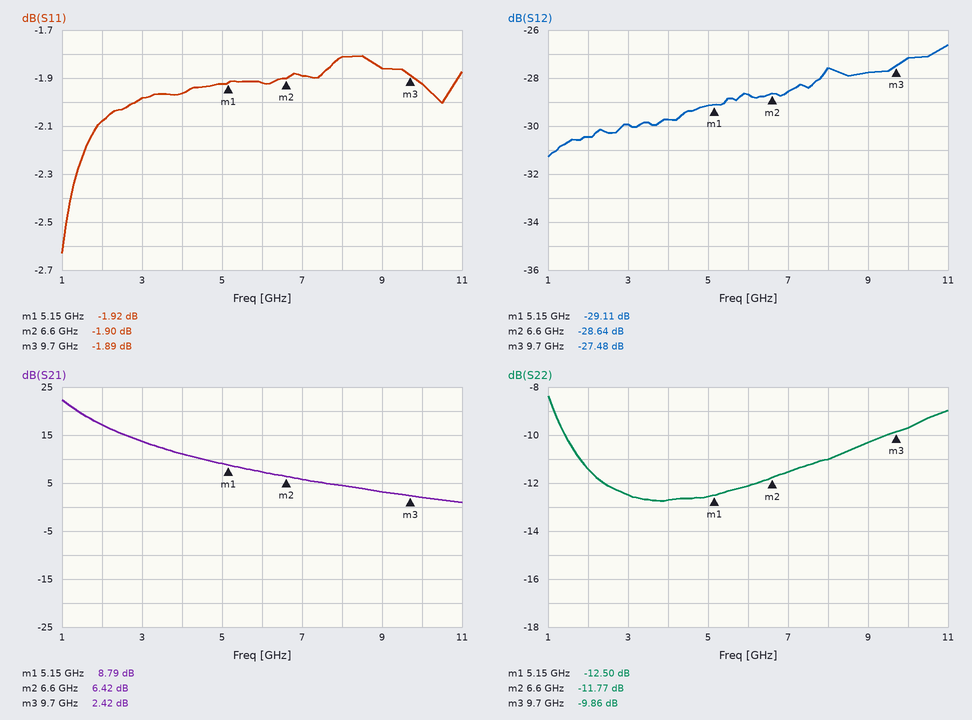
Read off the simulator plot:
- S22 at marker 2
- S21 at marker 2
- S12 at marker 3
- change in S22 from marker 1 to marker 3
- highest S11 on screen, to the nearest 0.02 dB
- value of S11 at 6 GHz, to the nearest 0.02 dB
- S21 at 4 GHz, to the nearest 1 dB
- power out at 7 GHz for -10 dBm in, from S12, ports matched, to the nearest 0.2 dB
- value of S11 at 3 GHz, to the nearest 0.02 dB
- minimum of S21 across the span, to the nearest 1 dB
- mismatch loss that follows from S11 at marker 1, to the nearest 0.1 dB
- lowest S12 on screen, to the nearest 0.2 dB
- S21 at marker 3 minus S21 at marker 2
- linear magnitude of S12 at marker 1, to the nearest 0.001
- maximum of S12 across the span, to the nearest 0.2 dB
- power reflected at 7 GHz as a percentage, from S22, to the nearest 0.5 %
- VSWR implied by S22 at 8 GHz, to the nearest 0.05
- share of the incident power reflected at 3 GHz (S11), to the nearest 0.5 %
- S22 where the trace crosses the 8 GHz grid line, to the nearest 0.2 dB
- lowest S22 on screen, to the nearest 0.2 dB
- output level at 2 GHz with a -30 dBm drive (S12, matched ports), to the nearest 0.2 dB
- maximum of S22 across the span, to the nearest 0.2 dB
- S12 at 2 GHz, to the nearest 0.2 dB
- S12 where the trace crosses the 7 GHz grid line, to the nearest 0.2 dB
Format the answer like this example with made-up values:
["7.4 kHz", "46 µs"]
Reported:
["-11.77 dB", "6.42 dB", "-27.48 dB", "2.64 dB", "-1.80 dB", "-1.92 dB", "11 dB", "-38.6 dBm", "-1.98 dB", "1 dB", "4.5 dB", "-31.2 dB", "-4.00 dB", "0.035", "-26.6 dB", "7.0 %", "1.80", "63.5 %", "-11.0 dB", "-12.8 dB", "-60.4 dBm", "-8.4 dB", "-30.4 dB", "-28.6 dB"]
